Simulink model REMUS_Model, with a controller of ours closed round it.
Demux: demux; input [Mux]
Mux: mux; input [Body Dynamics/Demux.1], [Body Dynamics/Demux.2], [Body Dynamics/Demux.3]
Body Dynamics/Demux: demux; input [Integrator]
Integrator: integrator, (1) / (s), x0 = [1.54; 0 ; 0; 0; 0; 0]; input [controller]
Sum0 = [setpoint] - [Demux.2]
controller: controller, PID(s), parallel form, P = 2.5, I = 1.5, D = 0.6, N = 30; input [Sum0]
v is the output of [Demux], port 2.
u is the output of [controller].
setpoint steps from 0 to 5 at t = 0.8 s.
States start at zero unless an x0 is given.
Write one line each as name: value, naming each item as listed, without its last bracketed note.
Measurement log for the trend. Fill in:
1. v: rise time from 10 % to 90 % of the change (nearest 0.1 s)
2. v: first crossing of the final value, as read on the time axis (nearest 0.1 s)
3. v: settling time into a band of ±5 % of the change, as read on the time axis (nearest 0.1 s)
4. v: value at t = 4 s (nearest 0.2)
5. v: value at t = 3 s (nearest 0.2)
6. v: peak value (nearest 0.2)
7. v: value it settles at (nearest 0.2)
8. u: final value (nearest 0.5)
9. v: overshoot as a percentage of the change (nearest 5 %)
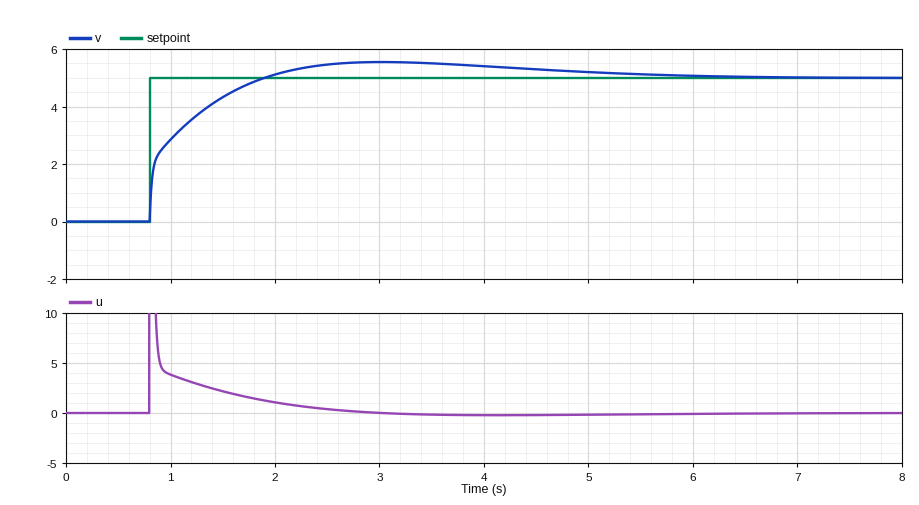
v: rise time from 10 % to 90 % of the change: 0.8 s
v: first crossing of the final value, as read on the time axis: 1.9 s
v: settling time into a band of ±5 % of the change, as read on the time axis: 4.7 s
v: value at t = 4 s: 5.4
v: value at t = 3 s: 5.6
v: peak value: 5.6
v: value it settles at: 5.0
u: final value: 0.0
v: overshoot as a percentage of the change: 10 %
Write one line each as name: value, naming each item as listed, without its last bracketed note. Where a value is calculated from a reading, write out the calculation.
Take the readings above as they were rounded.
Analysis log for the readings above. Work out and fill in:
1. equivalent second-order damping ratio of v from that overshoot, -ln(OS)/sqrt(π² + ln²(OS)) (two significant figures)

equivalent second-order damping ratio of v from that overshoot, -ln(OS)/sqrt(π² + ln²(OS)): ln(0.1) = -2.303; 2.303 / sqrt(9.870 + 5.302) = 0.59
